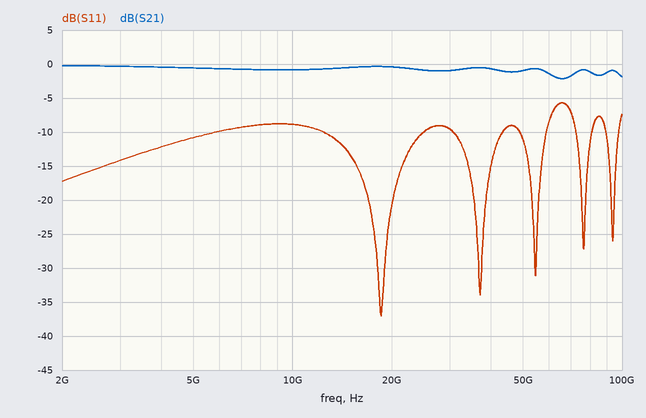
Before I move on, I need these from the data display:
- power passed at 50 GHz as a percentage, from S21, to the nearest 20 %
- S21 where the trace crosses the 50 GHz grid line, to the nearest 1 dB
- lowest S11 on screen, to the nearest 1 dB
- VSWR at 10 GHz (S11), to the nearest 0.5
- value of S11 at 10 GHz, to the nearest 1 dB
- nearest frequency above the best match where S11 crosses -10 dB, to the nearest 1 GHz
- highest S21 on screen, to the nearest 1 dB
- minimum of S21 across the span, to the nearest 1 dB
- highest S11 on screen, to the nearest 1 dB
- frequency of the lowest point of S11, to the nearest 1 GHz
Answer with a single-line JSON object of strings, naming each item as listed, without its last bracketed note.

{"power passed at 50 GHz as a percentage, from S21, to the nearest 20 %": "80 %", "S21 where the trace crosses the 50 GHz grid line, to the nearest 1 dB": "-1 dB", "lowest S11 on screen, to the nearest 1 dB": "-37 dB", "VSWR at 10 GHz (S11), to the nearest 0.5": "2.0", "value of S11 at 10 GHz, to the nearest 1 dB": "-9 dB", "nearest frequency above the best match where S11 crosses -10 dB, to the nearest 1 GHz": "25 GHz", "highest S21 on screen, to the nearest 1 dB": "0 dB", "minimum of S21 across the span, to the nearest 1 dB": "-2 dB", "highest S11 on screen, to the nearest 1 dB": "-6 dB", "frequency of the lowest point of S11, to the nearest 1 GHz": "19 GHz"}
